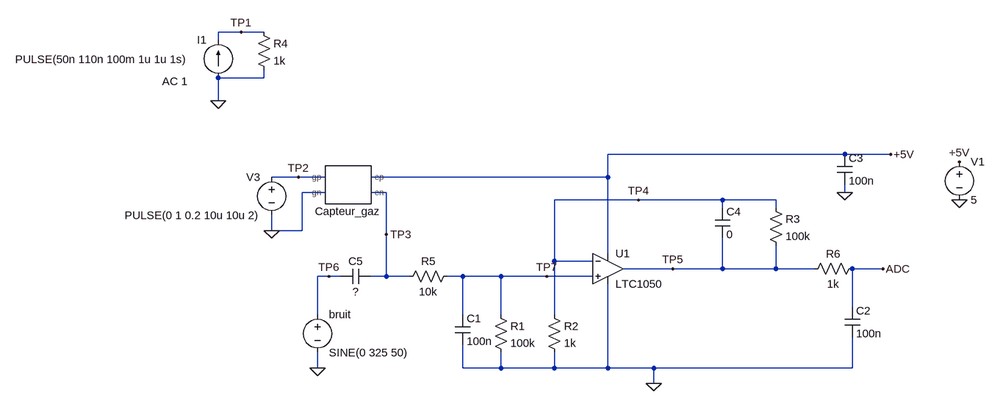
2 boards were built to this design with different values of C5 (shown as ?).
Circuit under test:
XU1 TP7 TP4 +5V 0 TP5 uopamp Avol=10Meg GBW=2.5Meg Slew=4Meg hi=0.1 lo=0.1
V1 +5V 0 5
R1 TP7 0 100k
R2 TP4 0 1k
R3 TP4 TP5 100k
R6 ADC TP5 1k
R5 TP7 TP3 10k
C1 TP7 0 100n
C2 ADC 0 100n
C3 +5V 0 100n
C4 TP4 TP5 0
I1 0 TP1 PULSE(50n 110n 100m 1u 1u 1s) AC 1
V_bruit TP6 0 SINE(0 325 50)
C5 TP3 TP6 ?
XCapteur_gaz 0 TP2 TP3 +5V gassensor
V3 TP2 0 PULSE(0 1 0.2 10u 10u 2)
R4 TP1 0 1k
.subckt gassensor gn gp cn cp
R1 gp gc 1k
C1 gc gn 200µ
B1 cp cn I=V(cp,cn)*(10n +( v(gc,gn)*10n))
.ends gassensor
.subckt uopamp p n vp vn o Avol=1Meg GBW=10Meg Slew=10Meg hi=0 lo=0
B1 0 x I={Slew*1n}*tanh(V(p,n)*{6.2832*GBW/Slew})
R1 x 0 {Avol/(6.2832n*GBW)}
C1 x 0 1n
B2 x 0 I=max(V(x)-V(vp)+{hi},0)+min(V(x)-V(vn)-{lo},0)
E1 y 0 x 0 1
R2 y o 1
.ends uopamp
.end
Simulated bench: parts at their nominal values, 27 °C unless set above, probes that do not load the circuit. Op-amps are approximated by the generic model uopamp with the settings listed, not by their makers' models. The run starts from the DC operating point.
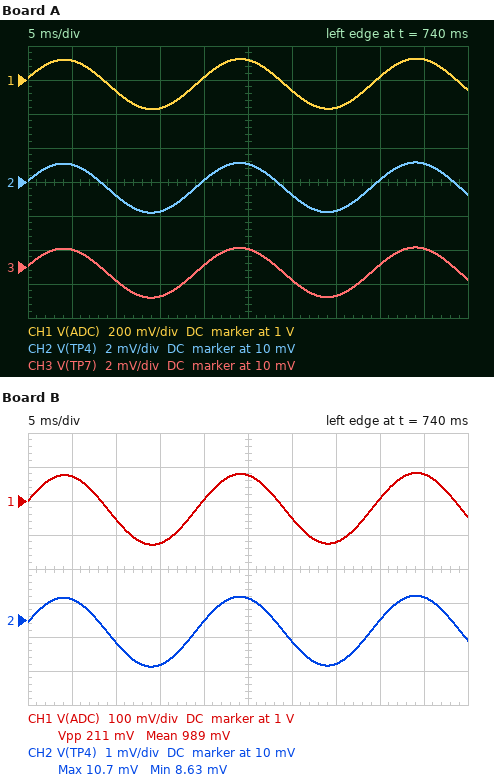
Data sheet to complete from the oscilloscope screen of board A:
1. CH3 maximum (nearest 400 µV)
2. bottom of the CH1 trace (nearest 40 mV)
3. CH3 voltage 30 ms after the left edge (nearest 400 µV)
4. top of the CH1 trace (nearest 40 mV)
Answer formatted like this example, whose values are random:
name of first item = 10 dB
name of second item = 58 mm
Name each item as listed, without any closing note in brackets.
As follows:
CH3 maximum = 11.2 mV
bottom of the CH1 trace = 840 mV
CH3 voltage 30 ms after the left edge = 9.2 mV
top of the CH1 trace = 1.12 V
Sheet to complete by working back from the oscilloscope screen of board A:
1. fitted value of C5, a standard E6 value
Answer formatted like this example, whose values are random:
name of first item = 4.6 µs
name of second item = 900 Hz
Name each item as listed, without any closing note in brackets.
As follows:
fitted value of C5, a standard E6 value = 470 fF
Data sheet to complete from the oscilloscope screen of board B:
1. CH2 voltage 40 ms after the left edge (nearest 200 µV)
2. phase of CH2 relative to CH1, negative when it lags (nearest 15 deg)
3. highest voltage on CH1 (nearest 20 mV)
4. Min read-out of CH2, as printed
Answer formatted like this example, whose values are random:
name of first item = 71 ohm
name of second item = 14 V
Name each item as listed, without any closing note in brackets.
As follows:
CH2 voltage 40 ms after the left edge = 10.0 mV
phase of CH2 relative to CH1, negative when it lags = 0 deg
highest voltage on CH1 = 1.08 V
Min read-out of CH2, as printed = 8.63 mV
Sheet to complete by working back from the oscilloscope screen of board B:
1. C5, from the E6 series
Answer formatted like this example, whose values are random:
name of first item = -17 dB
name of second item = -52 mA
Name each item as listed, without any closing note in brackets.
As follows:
C5, from the E6 series = 330 fF
